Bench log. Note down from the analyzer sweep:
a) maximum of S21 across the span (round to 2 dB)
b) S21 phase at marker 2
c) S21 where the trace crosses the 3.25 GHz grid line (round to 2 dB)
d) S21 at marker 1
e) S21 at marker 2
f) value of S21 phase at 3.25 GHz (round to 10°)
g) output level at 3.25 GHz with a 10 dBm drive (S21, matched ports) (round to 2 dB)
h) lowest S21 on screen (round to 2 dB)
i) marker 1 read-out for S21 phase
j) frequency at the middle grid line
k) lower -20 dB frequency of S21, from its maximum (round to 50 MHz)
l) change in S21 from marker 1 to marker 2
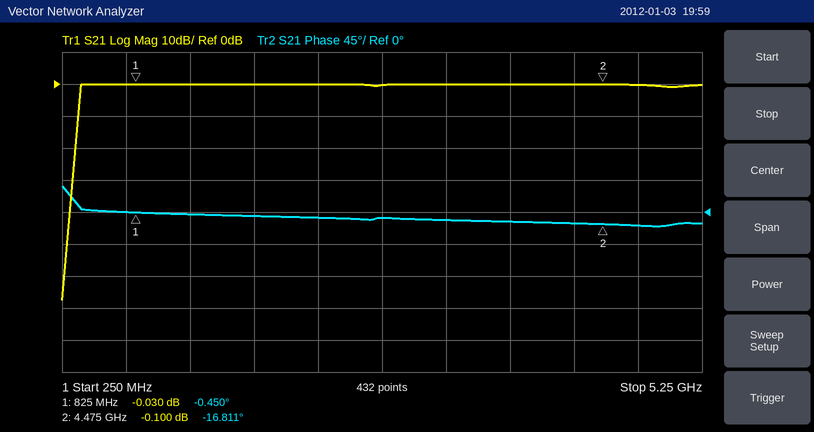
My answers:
0 dB
-16.811°
0 dB
-0.030 dB
-0.100 dB
-10°
10 dBm
-68 dB
-0.450°
2.75 GHz
350 MHz
-0.070 dB
